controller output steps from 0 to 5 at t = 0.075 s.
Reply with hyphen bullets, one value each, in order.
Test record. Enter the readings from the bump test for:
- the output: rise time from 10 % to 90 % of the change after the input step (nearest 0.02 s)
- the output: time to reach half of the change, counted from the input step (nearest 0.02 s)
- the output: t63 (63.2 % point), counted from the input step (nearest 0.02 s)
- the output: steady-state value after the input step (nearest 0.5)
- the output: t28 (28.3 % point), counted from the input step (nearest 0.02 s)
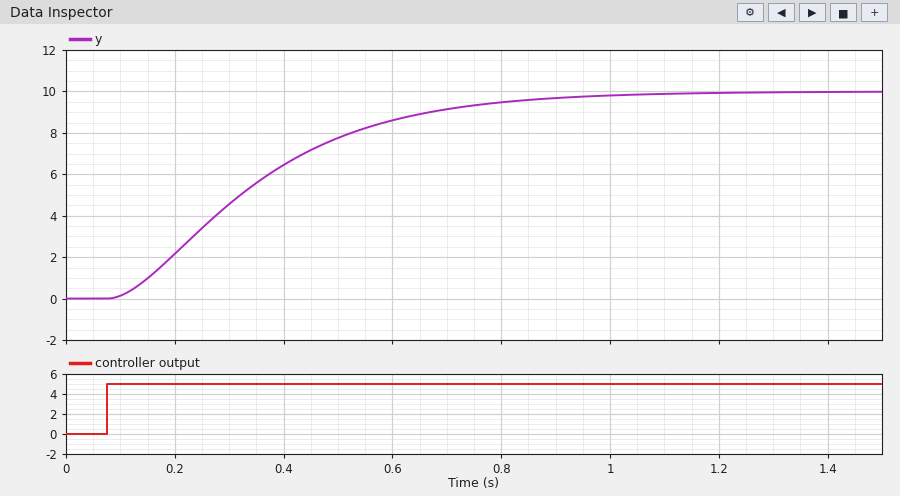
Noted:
- 0.52 s
- 0.24 s
- 0.32 s
- 10.0
- 0.16 s
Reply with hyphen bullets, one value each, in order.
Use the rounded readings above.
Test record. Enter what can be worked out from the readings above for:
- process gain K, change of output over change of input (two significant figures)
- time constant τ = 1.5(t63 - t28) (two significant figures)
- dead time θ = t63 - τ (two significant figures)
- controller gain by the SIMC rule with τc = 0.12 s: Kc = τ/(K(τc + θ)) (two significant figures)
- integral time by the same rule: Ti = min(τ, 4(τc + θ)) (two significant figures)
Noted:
- 2.0
- 0.24 s
- 0.080 s
- 0.60
- 0.24 s
